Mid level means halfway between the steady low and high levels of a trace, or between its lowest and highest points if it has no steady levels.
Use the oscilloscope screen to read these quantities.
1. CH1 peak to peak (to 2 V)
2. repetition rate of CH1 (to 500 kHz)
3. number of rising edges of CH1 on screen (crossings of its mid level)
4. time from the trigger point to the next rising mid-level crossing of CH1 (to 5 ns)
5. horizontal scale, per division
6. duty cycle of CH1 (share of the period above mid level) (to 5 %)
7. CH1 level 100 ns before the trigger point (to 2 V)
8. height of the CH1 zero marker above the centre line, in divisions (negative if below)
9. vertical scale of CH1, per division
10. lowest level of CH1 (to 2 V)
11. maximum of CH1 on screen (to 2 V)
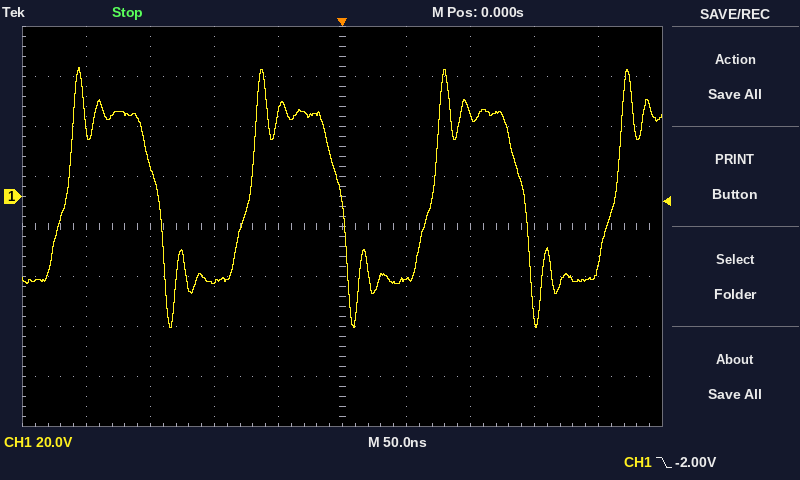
104 V
7.0 MHz
4
70 ns
50 ns
50 %
-34 V
+0.6 div
20 V
-52 V
52 V
